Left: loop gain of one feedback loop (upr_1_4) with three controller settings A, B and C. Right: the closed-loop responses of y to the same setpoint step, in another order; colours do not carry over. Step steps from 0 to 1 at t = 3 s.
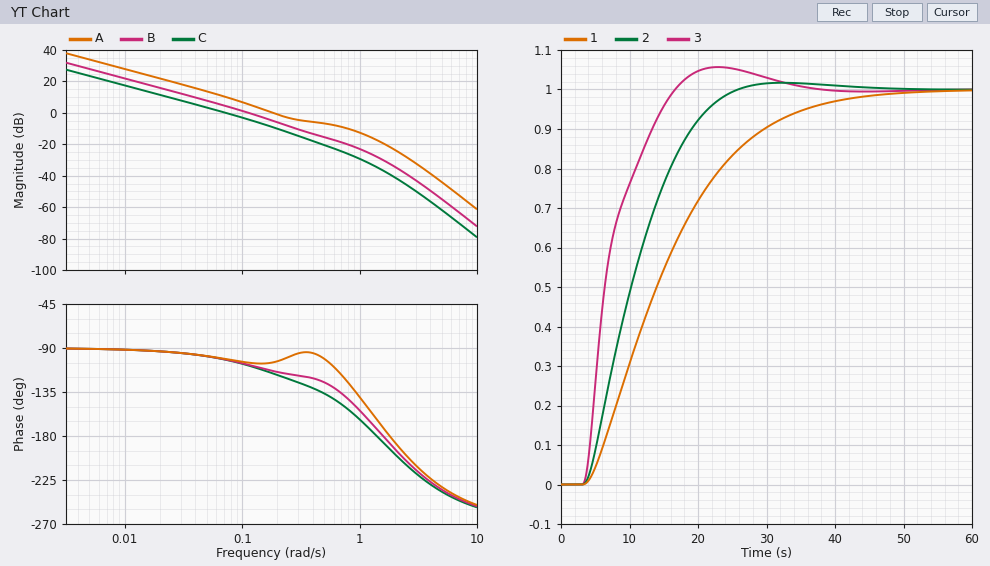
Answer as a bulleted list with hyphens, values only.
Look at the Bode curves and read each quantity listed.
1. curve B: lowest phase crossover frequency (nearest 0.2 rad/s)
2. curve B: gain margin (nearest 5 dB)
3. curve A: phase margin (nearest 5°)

- 1.6 rad/s
- 30 dB
- 75°
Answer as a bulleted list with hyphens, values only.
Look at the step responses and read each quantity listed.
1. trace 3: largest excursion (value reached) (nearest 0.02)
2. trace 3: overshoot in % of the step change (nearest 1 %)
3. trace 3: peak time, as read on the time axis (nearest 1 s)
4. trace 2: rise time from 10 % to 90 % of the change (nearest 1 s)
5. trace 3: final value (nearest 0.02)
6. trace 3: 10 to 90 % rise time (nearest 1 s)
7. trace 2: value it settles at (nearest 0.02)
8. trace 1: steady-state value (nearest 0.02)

- 1.06
- 6 %
- 23 s
- 14 s
- 1.00
- 9 s
- 1.00
- 1.00
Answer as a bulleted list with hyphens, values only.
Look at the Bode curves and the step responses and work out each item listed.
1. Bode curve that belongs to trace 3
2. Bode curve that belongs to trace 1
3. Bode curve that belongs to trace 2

- A
- C
- B
